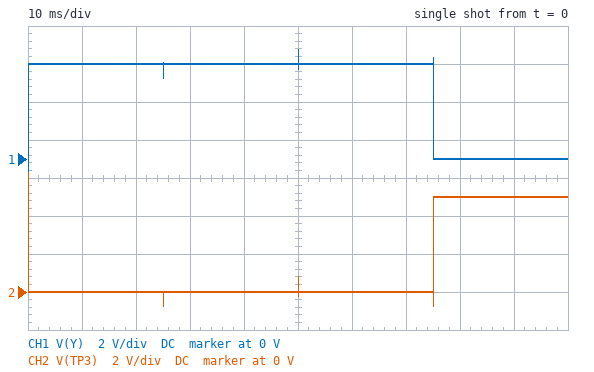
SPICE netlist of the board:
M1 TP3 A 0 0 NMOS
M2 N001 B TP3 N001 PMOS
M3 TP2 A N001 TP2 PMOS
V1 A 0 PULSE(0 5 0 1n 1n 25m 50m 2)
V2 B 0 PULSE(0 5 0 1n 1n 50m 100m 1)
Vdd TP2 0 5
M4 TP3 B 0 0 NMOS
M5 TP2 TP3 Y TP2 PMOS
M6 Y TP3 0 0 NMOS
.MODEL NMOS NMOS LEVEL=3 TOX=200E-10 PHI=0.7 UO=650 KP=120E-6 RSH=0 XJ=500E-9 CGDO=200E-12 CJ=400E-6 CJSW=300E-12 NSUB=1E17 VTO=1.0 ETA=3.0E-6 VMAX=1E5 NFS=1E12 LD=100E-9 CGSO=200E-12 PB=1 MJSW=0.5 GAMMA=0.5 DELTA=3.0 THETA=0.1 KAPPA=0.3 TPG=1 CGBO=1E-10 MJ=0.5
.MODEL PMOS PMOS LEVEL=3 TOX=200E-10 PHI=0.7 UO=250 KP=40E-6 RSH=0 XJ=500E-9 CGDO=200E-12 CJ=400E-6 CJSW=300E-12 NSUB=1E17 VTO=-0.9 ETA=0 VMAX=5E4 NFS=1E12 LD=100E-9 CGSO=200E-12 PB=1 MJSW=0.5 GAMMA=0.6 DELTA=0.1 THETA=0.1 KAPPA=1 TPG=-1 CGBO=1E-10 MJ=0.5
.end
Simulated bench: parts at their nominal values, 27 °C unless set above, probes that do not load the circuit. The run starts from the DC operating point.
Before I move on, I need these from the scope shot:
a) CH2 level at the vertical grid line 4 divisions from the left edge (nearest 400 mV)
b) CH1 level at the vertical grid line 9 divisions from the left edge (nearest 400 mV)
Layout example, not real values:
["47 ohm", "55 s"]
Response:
["0 V", "0 V"]
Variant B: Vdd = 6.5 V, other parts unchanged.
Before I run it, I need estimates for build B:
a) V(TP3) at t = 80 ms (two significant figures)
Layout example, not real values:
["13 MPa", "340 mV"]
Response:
["6.5 V"]
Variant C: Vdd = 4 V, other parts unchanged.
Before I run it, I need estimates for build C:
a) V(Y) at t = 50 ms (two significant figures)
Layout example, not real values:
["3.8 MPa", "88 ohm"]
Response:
["4.0 V"]
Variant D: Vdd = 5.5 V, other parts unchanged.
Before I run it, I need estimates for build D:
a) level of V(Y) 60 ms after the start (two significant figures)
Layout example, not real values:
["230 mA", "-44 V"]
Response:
["5.5 V"]
